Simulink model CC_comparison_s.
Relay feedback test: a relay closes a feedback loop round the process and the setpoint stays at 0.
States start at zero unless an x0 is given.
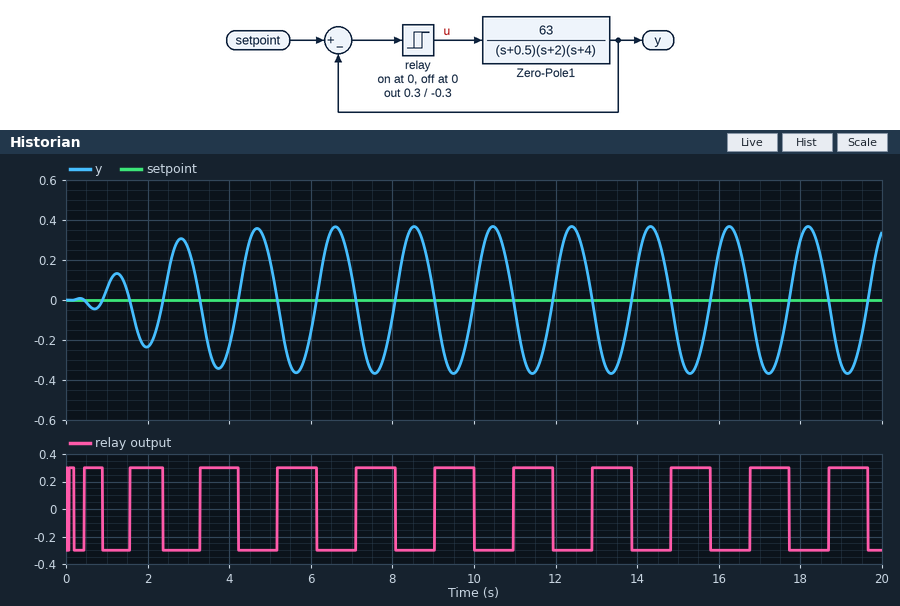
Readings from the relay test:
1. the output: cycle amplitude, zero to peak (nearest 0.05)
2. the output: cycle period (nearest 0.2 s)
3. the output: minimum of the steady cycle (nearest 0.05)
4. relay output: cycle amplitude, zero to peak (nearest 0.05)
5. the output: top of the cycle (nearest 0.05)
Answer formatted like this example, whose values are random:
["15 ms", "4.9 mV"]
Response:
["0.35", "2.0 s", "-0.35", "0.30", "0.35"]
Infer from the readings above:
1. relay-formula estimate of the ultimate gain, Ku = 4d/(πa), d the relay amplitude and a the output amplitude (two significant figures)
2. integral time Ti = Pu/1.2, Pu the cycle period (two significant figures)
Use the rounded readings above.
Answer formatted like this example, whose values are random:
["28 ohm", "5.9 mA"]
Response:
["1.1", "1.7 s"]
